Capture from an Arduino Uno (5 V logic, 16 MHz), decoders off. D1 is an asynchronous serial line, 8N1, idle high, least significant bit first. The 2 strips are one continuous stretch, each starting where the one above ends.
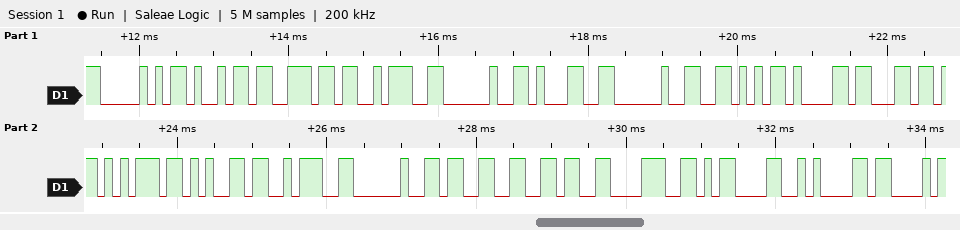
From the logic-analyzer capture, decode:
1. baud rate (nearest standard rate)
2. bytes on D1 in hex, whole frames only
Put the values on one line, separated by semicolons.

9600 baud; 0x50 0x69 0x6E 0x3A 0x20 0x31 0x20 0x56 0x61 0x6C 0x75 0x65 0x3A 0x20 0x33 0x36 0x38 0x0D 0x0A 0x43
